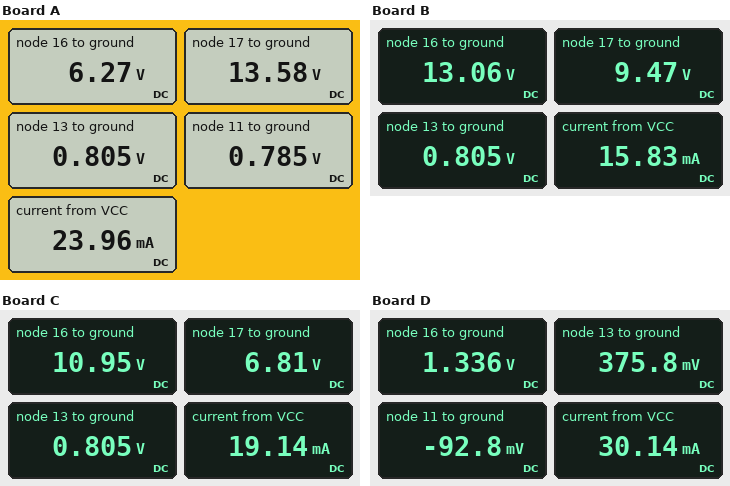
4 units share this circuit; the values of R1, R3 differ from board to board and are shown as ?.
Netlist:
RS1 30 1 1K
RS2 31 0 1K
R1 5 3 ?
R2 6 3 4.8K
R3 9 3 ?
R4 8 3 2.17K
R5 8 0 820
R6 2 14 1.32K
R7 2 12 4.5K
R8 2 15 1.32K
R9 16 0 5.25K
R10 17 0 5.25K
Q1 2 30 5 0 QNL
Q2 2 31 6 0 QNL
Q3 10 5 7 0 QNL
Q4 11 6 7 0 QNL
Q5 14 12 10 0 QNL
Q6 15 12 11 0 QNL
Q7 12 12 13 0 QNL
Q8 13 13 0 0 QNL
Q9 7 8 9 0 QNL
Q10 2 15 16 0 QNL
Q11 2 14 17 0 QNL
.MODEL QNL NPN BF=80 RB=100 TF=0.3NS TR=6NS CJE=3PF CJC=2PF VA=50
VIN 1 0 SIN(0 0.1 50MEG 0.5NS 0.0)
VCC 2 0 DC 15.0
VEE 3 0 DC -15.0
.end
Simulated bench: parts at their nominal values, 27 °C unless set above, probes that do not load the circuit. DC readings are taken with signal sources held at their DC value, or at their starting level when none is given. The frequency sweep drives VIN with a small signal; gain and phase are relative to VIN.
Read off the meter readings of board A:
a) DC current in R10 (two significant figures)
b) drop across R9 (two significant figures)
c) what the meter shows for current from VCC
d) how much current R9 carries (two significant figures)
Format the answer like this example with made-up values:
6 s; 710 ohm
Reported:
2.6 mA; 6.3 V; 23.96 mA; 1.2 mA
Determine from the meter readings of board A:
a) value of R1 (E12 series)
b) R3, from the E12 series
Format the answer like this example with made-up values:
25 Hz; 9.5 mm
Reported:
1.8 kΩ; 1.5 kΩ
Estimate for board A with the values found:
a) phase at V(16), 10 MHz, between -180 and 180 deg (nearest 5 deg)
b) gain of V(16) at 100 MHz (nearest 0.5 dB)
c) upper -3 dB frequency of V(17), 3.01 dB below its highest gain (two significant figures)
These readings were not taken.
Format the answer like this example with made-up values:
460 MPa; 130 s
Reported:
-20 deg; 9.5 dB; 48 MHz
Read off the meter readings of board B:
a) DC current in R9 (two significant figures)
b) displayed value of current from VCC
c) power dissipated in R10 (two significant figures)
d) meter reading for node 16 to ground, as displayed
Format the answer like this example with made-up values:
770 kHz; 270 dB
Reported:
2.5 mA; 15.83 mA; 17 mW; 13.06 V
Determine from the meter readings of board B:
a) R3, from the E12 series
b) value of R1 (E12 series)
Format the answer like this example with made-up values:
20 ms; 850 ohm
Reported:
2.2 kΩ; 12 kΩ
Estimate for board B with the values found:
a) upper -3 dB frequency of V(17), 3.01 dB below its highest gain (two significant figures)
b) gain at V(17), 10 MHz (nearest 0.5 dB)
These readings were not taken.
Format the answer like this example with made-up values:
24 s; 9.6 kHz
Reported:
45 MHz; 30.0 dB
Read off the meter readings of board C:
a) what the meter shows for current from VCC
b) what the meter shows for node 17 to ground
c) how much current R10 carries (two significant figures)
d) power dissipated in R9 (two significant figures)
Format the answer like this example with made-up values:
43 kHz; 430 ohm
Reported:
19.14 mA; 6.81 V; 1.3 mA; 23 mW
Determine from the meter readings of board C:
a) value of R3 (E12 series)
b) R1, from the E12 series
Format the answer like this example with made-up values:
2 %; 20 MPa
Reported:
1.2 kΩ; 8.2 kΩ
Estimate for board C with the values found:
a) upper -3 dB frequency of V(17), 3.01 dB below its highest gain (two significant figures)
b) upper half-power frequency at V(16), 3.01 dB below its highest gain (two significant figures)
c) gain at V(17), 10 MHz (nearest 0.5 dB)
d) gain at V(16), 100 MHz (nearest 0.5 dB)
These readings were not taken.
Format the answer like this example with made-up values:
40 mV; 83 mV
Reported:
31 MHz; 31 MHz; 37.0 dB; 11.0 dB
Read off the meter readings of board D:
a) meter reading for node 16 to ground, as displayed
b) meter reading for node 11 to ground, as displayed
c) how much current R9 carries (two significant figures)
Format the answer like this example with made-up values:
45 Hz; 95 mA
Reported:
1.336 V; -92.8 mV; 250 µA
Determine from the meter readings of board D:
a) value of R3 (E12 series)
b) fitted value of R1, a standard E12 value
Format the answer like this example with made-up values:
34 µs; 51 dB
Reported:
390 Ω; 6.8 kΩ
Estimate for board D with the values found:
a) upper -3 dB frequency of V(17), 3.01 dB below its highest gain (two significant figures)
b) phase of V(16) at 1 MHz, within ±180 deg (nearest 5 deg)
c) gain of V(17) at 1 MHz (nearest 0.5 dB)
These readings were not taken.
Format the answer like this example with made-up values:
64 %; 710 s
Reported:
19 MHz; -5 deg; 21.0 dB
